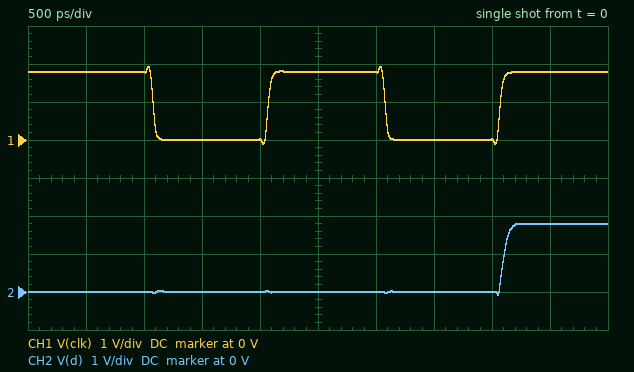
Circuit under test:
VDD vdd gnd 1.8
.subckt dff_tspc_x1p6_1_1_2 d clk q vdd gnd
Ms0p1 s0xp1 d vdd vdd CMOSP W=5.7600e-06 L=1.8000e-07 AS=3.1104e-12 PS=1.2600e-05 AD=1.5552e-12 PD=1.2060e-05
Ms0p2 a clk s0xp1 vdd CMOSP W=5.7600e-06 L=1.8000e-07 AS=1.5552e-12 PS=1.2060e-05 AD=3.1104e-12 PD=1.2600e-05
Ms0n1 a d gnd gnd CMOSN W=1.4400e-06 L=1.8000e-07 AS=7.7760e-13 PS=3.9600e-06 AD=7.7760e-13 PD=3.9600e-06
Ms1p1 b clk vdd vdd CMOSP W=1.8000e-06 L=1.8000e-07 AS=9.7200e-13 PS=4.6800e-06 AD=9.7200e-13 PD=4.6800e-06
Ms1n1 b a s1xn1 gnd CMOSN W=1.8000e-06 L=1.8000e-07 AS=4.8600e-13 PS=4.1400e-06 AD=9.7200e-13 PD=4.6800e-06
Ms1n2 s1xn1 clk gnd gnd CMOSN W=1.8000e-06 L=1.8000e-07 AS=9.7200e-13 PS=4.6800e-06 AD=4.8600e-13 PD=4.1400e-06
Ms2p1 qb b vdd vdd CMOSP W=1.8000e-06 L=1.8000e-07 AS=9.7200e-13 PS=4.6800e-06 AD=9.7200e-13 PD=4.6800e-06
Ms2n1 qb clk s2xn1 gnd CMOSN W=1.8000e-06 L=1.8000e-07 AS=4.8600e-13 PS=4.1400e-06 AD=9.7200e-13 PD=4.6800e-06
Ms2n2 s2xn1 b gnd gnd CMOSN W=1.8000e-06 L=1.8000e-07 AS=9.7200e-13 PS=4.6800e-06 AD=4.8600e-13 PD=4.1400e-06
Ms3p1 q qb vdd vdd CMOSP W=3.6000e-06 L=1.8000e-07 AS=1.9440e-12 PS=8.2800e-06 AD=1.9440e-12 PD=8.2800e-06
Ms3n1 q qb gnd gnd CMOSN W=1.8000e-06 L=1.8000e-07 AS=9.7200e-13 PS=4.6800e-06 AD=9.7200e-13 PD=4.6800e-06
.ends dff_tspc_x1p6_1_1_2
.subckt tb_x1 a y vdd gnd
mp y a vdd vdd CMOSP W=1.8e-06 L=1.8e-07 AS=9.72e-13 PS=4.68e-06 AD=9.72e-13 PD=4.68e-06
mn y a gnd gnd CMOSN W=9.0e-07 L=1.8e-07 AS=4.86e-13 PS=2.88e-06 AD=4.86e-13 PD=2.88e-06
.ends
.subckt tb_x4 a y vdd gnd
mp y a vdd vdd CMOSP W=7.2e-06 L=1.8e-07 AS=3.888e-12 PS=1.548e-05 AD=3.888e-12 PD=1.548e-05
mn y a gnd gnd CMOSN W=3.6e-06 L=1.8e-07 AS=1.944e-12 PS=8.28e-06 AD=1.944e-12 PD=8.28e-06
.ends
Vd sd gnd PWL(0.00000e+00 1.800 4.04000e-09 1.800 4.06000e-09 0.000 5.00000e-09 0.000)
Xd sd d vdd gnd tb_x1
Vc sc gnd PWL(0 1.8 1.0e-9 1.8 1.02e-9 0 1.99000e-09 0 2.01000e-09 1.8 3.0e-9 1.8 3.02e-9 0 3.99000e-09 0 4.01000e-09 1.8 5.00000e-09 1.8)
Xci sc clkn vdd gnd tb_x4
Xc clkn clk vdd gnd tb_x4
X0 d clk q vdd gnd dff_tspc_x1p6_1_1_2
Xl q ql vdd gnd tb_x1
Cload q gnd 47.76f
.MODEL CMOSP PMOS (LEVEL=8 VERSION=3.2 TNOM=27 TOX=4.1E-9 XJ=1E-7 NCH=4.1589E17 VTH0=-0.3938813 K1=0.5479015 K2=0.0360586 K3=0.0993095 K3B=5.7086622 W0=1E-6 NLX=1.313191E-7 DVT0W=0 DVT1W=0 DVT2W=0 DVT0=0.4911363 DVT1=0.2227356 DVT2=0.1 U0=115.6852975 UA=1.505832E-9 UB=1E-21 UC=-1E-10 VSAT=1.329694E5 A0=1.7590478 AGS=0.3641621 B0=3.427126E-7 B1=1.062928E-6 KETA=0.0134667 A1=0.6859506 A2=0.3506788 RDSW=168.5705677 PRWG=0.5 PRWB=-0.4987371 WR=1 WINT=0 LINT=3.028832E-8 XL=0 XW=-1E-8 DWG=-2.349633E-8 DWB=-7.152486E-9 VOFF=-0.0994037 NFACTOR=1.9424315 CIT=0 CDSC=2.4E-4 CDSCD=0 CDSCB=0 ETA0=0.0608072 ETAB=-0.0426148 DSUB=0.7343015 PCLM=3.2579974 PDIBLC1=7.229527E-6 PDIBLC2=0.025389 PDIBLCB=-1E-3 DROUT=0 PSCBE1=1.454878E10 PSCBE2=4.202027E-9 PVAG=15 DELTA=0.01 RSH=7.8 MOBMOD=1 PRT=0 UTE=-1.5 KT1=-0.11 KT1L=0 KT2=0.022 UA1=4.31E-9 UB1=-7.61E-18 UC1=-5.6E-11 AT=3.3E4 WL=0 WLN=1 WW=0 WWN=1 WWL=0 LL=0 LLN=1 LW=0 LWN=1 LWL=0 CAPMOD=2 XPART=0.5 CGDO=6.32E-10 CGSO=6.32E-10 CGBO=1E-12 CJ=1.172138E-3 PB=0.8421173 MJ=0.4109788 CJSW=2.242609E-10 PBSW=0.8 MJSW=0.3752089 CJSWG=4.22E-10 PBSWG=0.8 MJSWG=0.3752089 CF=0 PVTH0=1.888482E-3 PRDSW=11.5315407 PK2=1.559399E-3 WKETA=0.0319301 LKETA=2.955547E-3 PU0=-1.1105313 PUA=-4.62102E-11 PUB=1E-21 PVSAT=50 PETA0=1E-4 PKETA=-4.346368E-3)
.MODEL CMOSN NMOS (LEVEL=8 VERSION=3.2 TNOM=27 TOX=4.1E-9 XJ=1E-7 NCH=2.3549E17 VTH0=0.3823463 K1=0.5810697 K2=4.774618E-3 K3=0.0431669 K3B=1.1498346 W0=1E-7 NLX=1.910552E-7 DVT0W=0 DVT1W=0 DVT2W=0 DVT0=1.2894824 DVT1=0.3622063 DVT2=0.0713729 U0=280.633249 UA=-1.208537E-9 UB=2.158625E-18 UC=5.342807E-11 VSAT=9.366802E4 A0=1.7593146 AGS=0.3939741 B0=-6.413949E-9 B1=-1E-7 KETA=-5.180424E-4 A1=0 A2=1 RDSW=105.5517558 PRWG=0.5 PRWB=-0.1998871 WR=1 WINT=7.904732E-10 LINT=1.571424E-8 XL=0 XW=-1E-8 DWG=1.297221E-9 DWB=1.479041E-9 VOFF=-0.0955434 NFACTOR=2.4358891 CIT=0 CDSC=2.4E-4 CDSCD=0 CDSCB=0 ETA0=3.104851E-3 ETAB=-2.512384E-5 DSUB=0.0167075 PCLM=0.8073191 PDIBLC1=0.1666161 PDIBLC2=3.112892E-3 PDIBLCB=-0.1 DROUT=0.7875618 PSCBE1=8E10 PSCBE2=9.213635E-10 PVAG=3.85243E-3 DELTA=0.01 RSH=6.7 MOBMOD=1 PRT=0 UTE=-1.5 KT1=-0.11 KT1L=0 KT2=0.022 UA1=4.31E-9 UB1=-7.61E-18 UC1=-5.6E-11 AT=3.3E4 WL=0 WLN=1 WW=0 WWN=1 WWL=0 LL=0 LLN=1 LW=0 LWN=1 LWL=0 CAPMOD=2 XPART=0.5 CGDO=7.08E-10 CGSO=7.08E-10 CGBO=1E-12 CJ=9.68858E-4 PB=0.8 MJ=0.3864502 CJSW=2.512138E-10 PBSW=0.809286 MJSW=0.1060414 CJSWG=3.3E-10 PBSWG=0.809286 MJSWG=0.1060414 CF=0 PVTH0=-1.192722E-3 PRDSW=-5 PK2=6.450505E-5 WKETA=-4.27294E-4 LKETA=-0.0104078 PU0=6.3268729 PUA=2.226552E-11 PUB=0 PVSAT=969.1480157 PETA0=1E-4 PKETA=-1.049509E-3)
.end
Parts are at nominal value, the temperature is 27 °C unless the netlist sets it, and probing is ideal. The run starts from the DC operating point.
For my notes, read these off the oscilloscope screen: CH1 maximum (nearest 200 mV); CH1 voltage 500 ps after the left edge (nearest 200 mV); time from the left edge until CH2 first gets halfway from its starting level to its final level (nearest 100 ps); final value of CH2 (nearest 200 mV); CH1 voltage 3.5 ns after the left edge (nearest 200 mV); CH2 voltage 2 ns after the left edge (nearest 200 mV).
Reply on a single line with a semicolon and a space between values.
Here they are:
2.0 V; 1.8 V; 4.1 ns; 1.8 V; 0 V; 0 V
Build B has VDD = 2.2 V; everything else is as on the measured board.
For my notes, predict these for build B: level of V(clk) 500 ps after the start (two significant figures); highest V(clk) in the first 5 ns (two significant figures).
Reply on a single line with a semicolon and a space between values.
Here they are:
2.2 V; 2.3 V
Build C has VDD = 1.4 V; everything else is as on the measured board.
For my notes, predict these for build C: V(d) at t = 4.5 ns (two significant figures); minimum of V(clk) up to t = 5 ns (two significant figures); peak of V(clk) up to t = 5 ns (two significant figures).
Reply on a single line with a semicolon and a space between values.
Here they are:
1.4 V; -140 mV; 1.5 V
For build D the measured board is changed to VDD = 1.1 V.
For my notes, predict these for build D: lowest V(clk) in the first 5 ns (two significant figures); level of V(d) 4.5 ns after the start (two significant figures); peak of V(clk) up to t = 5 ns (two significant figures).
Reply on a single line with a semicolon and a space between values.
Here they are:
-170 mV; 1.1 V; 1.2 V
